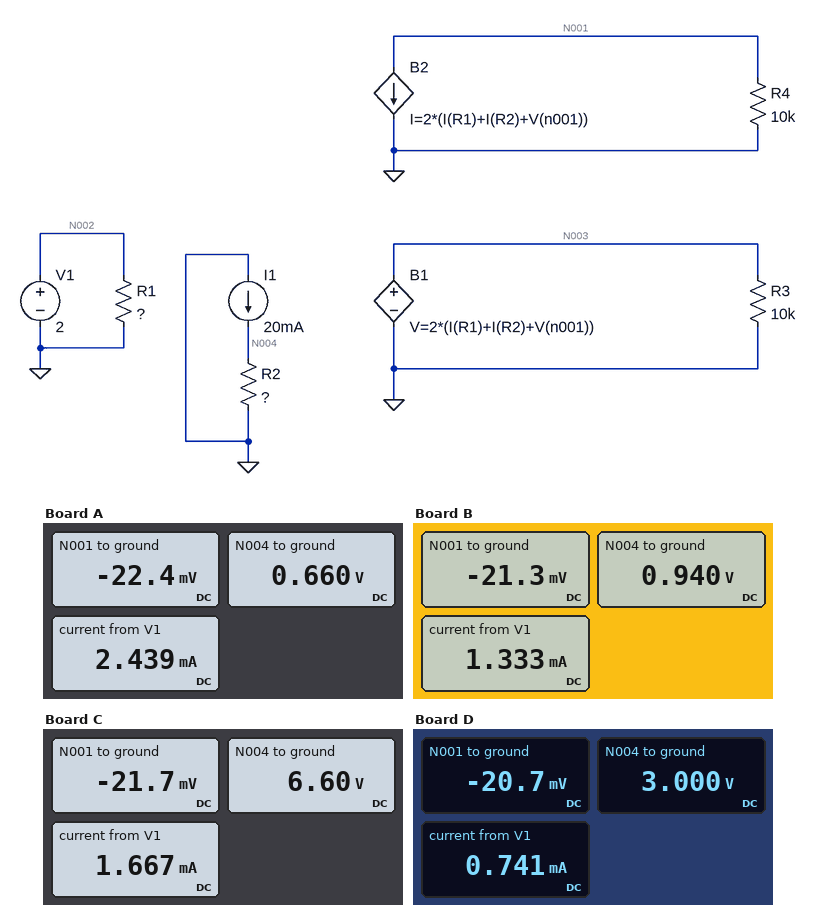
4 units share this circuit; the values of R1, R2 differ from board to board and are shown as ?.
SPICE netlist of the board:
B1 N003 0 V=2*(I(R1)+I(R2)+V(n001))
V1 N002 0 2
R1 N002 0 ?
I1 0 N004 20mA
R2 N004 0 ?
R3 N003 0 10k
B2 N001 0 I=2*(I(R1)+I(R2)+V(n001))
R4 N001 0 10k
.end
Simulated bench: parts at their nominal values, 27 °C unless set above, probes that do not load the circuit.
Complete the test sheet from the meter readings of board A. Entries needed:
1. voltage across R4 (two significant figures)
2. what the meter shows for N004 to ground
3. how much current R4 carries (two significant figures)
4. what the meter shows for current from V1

22 mV
0.660 V
2.2 µA
2.439 mA
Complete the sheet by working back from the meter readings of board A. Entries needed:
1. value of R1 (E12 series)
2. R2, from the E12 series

820 Ω
33 Ω
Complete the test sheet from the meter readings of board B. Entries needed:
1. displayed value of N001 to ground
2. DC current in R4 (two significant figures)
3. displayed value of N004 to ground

-21.3 mV
2.1 µA
0.940 V
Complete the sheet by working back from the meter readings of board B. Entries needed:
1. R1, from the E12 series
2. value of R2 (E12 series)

1.5 kΩ
47 Ω
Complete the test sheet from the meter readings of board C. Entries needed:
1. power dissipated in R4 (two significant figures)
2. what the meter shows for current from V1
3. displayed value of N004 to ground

47 nW
1.667 mA
6.60 V
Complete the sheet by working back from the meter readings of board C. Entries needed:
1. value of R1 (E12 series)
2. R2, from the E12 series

1.2 kΩ
330 Ω
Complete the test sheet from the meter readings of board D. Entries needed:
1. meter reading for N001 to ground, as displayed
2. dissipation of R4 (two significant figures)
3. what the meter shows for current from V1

-20.7 mV
43 nW
0.741 mA
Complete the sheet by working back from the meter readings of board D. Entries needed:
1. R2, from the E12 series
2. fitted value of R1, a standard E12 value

150 Ω
2.7 kΩ
